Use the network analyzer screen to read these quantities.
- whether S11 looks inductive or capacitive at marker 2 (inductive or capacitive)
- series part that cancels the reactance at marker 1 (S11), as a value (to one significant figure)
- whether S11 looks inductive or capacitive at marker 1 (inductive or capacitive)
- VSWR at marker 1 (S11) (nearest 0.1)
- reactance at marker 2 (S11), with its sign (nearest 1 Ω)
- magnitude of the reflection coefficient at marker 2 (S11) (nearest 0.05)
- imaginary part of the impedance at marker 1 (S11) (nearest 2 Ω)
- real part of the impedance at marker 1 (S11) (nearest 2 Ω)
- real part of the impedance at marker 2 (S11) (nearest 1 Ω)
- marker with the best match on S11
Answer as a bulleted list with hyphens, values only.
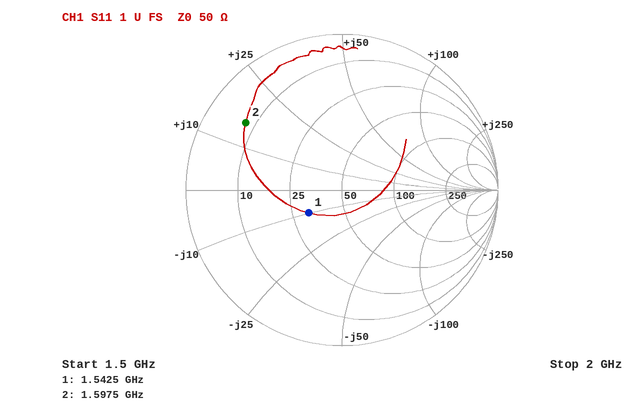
- inductive
- 1 nH
- capacitive
- 1.7
- +15 Ω
- 0.75
- -10 Ω
- 32 Ω
- 8 Ω
- marker 1
